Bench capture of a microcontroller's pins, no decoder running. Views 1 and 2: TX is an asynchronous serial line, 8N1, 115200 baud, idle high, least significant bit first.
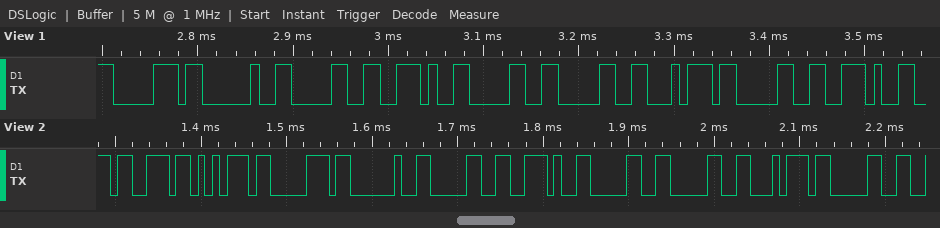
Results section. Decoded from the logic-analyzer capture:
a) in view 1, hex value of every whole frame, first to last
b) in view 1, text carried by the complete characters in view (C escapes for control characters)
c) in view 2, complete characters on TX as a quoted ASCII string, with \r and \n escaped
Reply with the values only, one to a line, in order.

0x70 0x20 0x30 0x2E 0x30 0x30 0x74 0x30 0x2E
"p 0.00t0."
"sup 0.00t0"
